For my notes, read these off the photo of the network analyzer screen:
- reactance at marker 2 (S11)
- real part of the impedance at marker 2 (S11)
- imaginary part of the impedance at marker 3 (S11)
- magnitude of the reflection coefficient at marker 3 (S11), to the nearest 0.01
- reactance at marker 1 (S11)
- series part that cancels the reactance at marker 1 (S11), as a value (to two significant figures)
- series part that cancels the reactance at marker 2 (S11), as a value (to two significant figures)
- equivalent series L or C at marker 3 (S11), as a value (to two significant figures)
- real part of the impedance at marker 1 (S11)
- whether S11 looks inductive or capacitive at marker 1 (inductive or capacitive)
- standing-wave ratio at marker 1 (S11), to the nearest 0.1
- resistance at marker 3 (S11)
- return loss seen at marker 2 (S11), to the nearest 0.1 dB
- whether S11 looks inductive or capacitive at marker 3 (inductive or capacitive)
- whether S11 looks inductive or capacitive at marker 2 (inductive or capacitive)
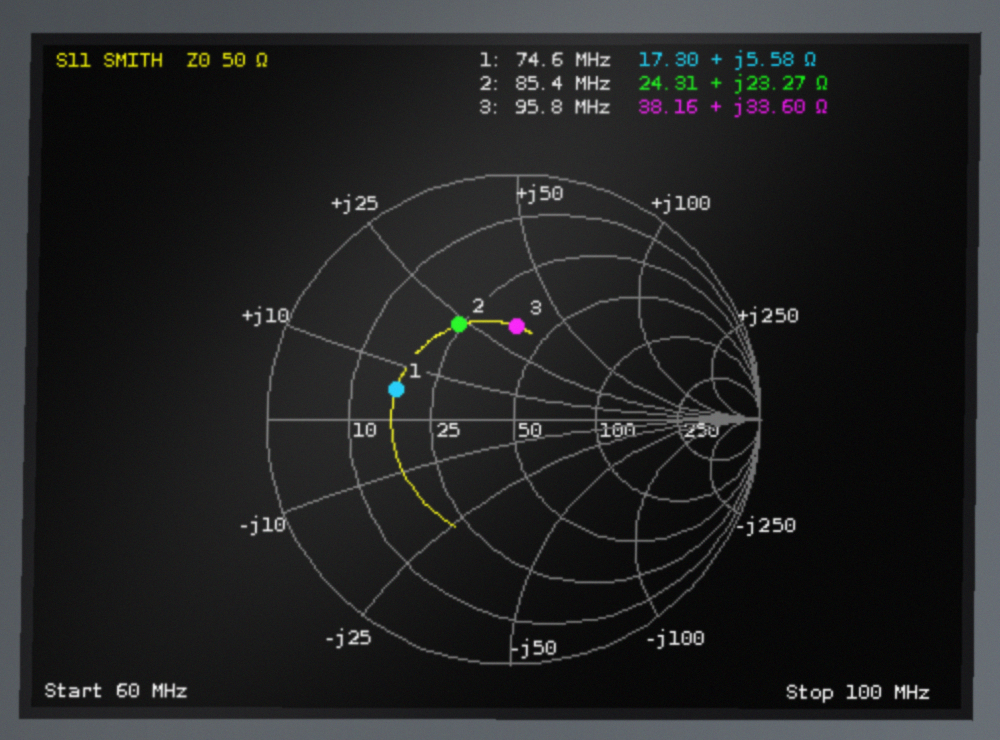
+23.27 Ω
24.31 Ω
+33.60 Ω
0.38
+5.58 Ω
380 pF
80 pF
56 nH
17.30 Ω
inductive
2.9
38.16 Ω
7.0 dB
inductive
inductive
